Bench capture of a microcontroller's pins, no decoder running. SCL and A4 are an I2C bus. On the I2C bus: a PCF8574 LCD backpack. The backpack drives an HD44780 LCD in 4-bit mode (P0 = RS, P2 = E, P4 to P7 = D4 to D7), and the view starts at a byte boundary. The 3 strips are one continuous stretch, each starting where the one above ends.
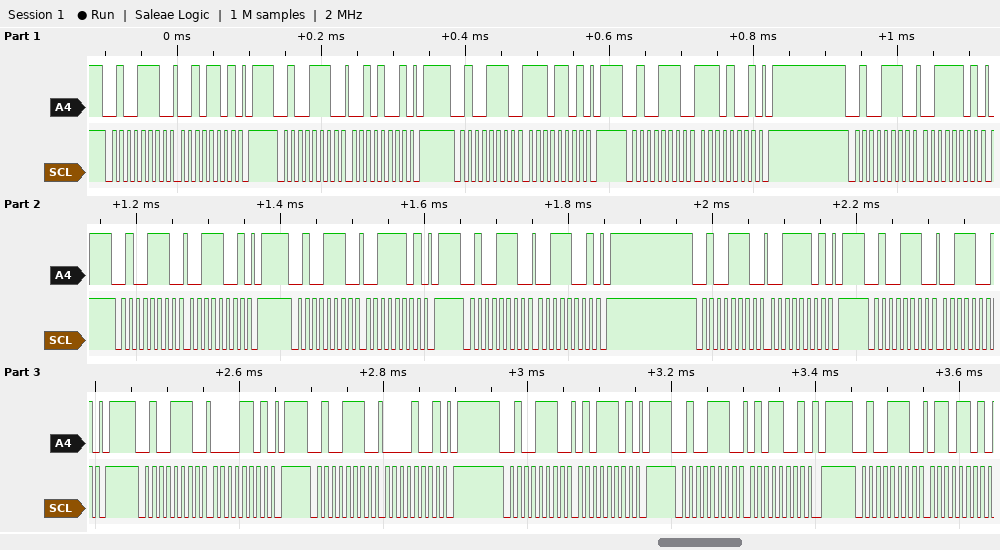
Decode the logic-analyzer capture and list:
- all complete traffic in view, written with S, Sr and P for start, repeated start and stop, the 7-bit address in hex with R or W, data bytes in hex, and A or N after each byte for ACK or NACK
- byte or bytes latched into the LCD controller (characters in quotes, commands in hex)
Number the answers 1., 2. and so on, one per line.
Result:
1. S 27W A 2D A P S 27W A 29 A P S 27W A ED A P S 27W A E9 A P S 27W A 3D A P S 27W A 39 A P S 27W A 3D A P S 27W A 39 A P S 27W A 3D A P S 27W A 39 A P S 27W A 0D A P S 27W A 09 A P S 27W A 5D A P S 27W A 59 A P S 27W A 6D A
2. '.' '3' '0'
